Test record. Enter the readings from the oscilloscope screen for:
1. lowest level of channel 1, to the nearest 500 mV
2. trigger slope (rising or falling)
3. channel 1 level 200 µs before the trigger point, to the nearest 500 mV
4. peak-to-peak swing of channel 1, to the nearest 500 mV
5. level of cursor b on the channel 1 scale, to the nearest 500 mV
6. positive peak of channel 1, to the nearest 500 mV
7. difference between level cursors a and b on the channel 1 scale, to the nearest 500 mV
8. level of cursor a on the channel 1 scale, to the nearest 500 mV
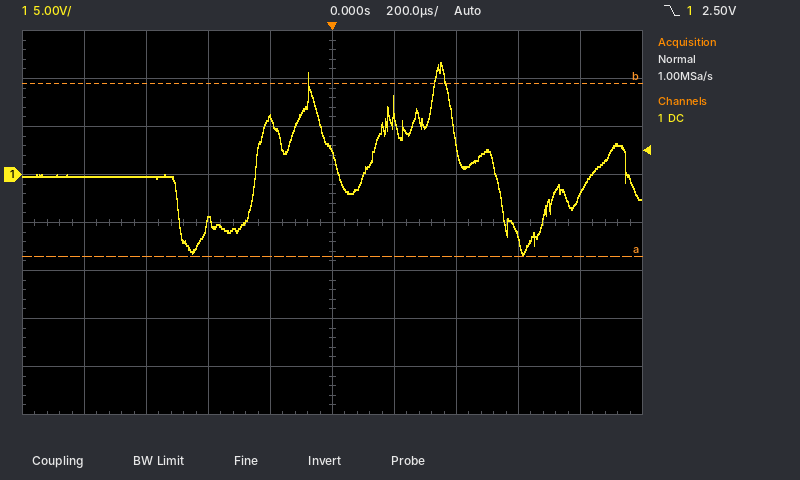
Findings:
-8.5 V
falling
6.0 V
20.0 V
9.5 V
11.5 V
18.0 V
-8.5 V
